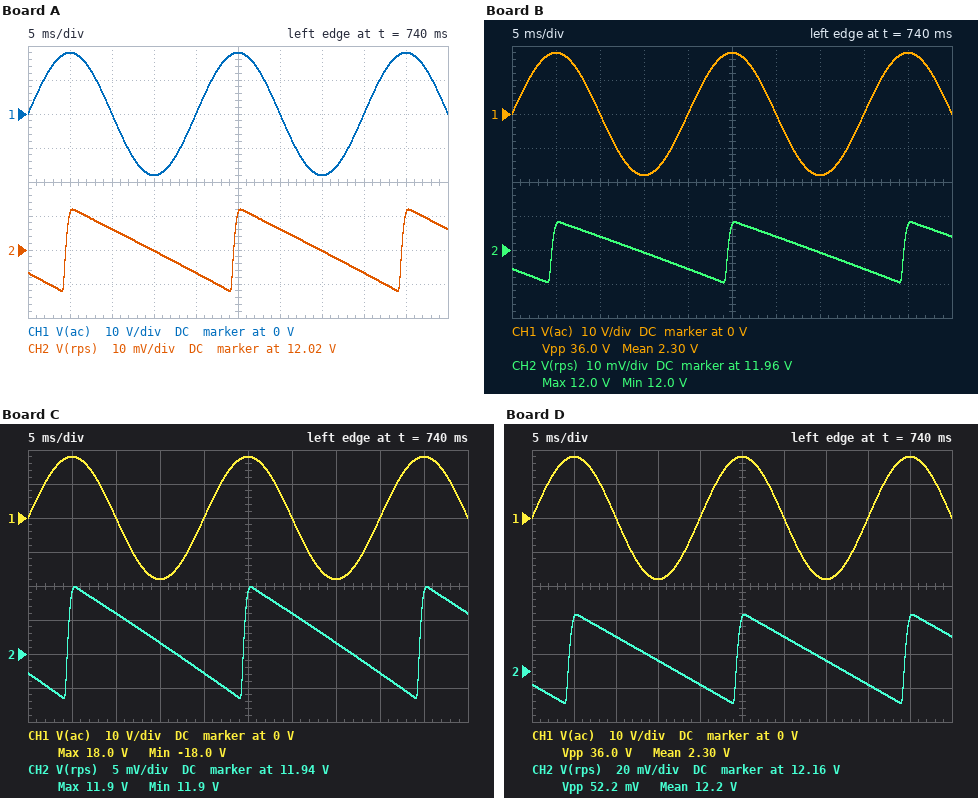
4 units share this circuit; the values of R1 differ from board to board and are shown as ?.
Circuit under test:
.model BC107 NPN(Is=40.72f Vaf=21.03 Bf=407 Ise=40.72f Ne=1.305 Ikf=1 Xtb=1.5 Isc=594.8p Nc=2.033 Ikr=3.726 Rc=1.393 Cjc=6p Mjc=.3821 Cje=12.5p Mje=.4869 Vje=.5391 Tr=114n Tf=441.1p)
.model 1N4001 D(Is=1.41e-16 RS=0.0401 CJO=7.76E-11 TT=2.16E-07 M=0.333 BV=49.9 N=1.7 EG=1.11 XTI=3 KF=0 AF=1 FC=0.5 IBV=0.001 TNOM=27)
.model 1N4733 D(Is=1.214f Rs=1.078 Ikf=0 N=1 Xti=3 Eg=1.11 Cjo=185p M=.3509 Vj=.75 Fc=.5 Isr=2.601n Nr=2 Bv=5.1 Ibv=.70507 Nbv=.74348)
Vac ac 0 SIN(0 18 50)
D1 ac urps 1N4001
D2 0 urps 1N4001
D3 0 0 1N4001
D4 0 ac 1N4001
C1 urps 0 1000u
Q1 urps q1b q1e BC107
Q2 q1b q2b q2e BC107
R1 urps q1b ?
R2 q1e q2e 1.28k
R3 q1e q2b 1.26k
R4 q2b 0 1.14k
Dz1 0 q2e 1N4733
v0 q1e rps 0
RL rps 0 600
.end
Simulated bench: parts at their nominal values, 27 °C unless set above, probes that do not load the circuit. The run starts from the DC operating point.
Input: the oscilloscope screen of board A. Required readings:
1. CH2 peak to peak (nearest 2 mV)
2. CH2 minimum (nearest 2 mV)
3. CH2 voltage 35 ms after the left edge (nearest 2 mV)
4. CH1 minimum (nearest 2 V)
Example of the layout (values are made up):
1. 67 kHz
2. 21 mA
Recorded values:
1. 24 mV
2. 12.008 V
3. 12.020 V
4. -18 V
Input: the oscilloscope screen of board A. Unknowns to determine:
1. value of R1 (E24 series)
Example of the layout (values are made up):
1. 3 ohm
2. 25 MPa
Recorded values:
1. 510 Ω
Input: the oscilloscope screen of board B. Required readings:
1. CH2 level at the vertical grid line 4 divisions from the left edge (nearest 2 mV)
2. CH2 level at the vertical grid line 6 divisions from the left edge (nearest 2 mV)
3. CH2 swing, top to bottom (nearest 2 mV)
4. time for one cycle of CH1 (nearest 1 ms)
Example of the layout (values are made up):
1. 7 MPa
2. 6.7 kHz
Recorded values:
1. 11.954 V
2. 11.964 V
3. 18 mV
4. 20 ms
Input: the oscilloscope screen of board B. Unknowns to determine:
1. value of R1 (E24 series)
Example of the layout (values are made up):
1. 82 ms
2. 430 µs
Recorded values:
1. 910 Ω
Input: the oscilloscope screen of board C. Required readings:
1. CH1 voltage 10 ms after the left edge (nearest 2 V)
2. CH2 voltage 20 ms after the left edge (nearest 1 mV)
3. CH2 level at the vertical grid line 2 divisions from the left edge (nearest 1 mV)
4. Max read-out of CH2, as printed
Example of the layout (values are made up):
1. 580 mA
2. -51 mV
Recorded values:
1. 0 V
2. 11.937 V
3. 11.946 V
4. 11.9 V
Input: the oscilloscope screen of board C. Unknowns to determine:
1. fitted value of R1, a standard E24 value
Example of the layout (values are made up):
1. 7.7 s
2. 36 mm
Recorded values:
1. 1.1 kΩ
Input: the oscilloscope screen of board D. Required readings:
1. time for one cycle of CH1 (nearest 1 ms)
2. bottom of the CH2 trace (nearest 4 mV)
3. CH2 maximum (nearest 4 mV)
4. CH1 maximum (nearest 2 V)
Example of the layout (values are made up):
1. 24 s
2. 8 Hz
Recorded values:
1. 20 ms
2. 12.140 V
3. 12.192 V
4. 18 V
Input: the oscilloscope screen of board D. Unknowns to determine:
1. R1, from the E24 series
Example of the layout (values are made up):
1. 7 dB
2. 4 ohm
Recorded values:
1. 180 Ω
